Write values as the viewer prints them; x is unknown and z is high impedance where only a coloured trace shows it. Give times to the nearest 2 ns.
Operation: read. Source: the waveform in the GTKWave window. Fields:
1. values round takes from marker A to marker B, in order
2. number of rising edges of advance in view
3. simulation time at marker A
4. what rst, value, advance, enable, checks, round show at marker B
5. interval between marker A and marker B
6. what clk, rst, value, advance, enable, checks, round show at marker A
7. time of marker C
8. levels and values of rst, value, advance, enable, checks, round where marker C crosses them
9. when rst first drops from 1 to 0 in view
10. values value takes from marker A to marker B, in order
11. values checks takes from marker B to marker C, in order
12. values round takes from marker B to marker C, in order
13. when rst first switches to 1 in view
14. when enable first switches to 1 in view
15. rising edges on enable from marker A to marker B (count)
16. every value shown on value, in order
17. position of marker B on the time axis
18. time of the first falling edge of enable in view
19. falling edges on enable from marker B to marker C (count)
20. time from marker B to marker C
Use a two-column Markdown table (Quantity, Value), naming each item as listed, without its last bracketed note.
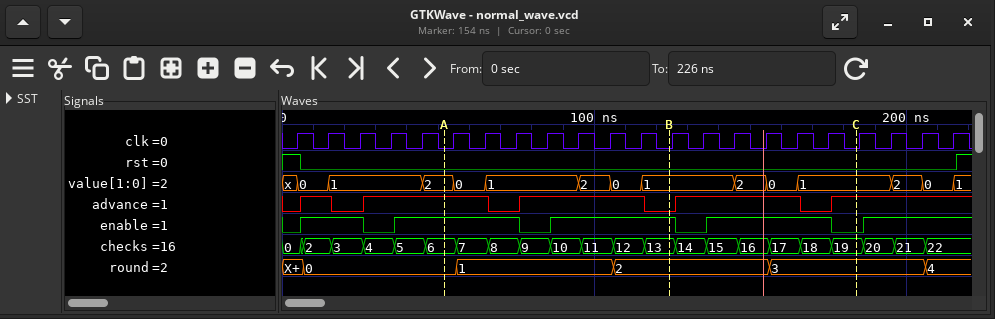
| Quantity | Value |
|---|---|
| values round takes from marker A to marker B, in order | 0, 1, 2 |
| number of rising edges of advance in view | 5 |
| simulation time at marker A | 52 ns |
| what rst, value, advance, enable, checks, round show at marker B | rst=0, value=1, advance=0, enable=1, checks=13, round=2 |
| interval between marker A and marker B | 72 ns |
| what clk, rst, value, advance, enable, checks, round show at marker A | clk=0, rst=0, value=2, advance=1, enable=1, checks=6, round=0 |
| time of marker C | 184 ns |
| levels and values of rst, value, advance, enable, checks, round where marker C crosses them | rst=0, value=1, advance=1, enable=0, checks=19, round=3 |
| when rst first drops from 1 to 0 in view | 6 ns |
| values value takes from marker A to marker B, in order | 2, 0, 1, 2, 0, 1 |
| values checks takes from marker B to marker C, in order | 13, 14, 15, 16, 17, 18, 19 |
| values round takes from marker B to marker C, in order | 2, 3 |
| when rst first switches to 1 in view | 216 ns |
| when enable first switches to 1 in view | 6 ns |
| rising edges on enable from marker A to marker B | 1 |
| every value shown on value, in order | x, 0, 1, 2, 0, 1, 2, 0, 1, 2, 0, 1, 2, 0, 1 |
| position of marker B on the time axis | 124 ns |
| time of the first falling edge of enable in view | 26 ns |
| falling edges on enable from marker B to marker C | 2 |
| time from marker B to marker C | 60 ns |
